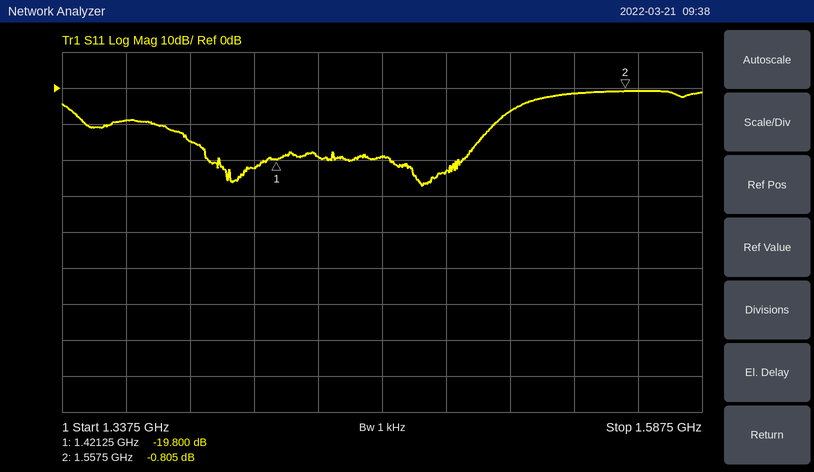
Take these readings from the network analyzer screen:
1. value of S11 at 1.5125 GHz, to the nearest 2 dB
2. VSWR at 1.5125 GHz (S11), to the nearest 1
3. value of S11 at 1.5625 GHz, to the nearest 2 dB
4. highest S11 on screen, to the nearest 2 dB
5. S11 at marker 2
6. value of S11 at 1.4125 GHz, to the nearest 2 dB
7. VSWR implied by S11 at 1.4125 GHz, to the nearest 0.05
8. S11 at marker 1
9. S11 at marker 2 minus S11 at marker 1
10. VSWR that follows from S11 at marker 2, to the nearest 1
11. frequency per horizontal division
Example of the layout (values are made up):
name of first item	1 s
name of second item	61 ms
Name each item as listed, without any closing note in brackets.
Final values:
value of S11 at 1.5125 GHz, to the nearest 2 dB	-6 dB
VSWR at 1.5125 GHz (S11), to the nearest 1	3
value of S11 at 1.5625 GHz, to the nearest 2 dB	0 dB
highest S11 on screen, to the nearest 2 dB	0 dB
S11 at marker 2	-0.805 dB
value of S11 at 1.4125 GHz, to the nearest 2 dB	-22 dB
VSWR implied by S11 at 1.4125 GHz, to the nearest 0.05	1.15
S11 at marker 1	-19.800 dB
S11 at marker 2 minus S11 at marker 1	18.995 dB
VSWR that follows from S11 at marker 2, to the nearest 1	22
frequency per horizontal division	25 MHz
